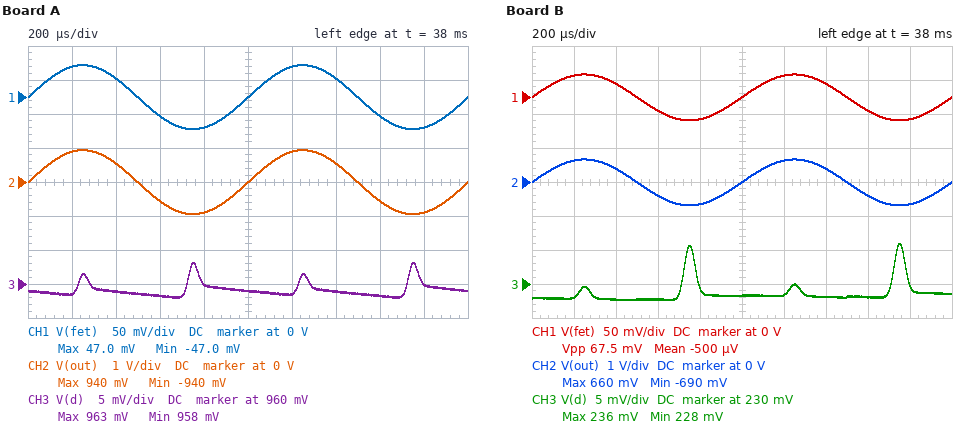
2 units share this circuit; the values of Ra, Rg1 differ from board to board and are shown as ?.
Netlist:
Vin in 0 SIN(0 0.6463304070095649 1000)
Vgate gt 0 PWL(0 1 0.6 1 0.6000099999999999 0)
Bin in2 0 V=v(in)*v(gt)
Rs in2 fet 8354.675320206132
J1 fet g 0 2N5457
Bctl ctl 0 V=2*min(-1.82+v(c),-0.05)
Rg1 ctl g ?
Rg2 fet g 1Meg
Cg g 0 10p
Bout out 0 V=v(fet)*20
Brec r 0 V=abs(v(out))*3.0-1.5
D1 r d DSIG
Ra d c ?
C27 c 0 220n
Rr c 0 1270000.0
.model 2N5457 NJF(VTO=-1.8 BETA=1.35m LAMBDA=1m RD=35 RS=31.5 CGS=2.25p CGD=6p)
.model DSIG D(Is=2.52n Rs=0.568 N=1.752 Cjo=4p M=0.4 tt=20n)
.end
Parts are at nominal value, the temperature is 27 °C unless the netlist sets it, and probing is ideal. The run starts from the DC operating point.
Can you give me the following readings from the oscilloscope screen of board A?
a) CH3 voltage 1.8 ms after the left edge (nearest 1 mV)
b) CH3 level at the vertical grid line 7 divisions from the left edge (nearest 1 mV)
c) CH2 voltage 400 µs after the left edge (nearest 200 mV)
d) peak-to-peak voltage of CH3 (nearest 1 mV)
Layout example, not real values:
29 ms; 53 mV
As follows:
960 mV; 959 mV; 600 mV; 5 mV
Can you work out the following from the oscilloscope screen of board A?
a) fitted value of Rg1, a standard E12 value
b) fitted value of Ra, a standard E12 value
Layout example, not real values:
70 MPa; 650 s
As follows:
470 kΩ; 470 Ω
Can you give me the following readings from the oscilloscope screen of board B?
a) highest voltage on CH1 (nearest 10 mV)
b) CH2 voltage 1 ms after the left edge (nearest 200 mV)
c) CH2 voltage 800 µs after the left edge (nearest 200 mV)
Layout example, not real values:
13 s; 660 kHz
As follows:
30 mV; 0 V; -600 mV
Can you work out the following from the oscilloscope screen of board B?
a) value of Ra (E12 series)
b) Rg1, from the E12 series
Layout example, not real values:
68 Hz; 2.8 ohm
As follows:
2.2 kΩ; 2.7 MΩ
